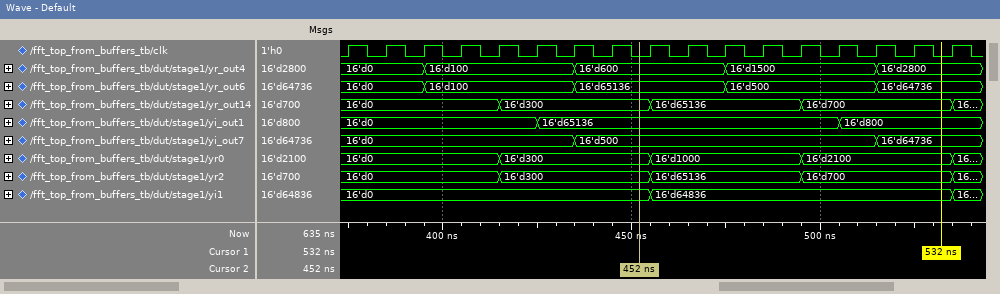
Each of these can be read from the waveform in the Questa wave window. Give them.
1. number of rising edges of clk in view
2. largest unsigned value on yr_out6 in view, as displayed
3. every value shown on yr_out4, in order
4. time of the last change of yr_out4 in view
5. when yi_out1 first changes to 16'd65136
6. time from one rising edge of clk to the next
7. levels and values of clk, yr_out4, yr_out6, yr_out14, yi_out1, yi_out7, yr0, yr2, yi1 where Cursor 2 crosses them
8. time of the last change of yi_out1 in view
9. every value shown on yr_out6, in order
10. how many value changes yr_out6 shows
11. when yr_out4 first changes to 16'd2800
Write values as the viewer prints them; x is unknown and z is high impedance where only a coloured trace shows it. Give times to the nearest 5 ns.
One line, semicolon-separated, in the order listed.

17; 16'd65136; 16'd0, 16'd100, 16'd600, 16'd1500, 16'd2800; 515 ns; 425 ns; 10 ns; clk=0, yr_out4=16'd600, yr_out6=16'd65136, yr_out14=16'd300, yi_out1=16'd65136, yi_out7=16'd500, yr0=16'd300, yr2=16'd300, yi1=16'd0; 505 ns; 16'd0, 16'd100, 16'd65136, 16'd500, 16'd64736; 4; 515 ns
